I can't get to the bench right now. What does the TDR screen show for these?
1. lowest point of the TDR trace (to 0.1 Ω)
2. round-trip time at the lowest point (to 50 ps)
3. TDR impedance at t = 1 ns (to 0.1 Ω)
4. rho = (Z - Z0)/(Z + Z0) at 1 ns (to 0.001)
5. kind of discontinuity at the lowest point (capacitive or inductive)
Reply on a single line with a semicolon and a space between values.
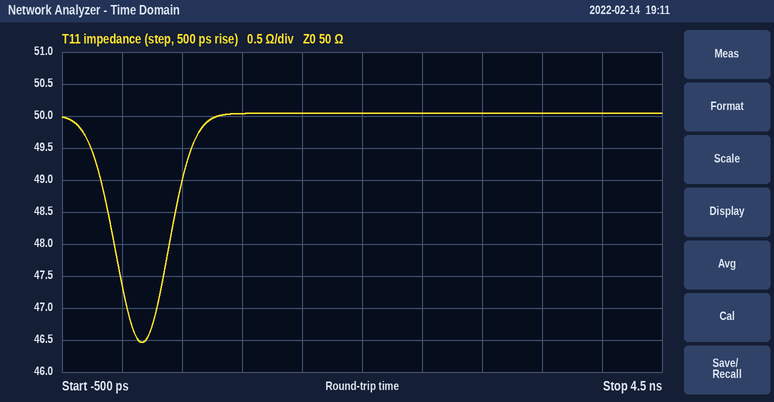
46.5 Ω; 150 ps; 50.0 Ω; 0.000; capacitive
